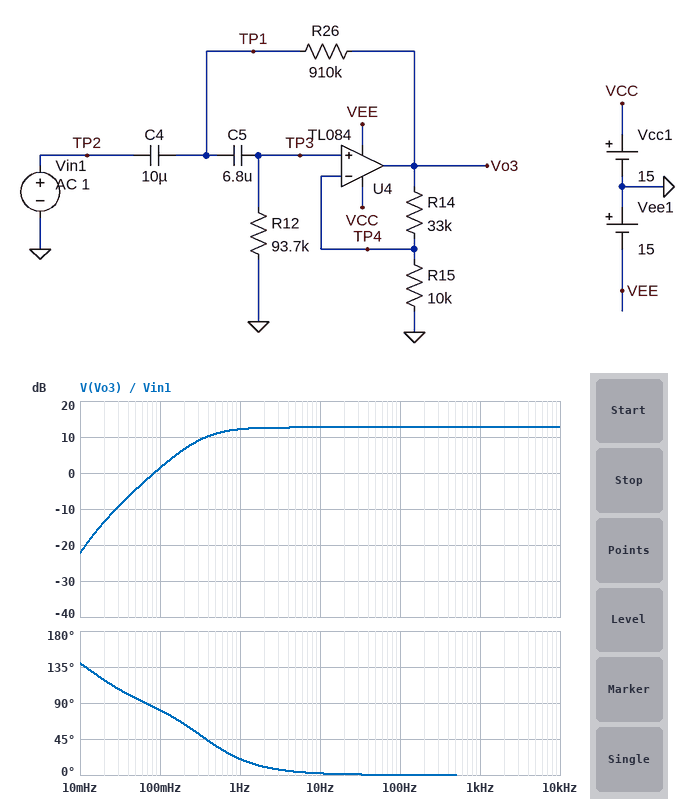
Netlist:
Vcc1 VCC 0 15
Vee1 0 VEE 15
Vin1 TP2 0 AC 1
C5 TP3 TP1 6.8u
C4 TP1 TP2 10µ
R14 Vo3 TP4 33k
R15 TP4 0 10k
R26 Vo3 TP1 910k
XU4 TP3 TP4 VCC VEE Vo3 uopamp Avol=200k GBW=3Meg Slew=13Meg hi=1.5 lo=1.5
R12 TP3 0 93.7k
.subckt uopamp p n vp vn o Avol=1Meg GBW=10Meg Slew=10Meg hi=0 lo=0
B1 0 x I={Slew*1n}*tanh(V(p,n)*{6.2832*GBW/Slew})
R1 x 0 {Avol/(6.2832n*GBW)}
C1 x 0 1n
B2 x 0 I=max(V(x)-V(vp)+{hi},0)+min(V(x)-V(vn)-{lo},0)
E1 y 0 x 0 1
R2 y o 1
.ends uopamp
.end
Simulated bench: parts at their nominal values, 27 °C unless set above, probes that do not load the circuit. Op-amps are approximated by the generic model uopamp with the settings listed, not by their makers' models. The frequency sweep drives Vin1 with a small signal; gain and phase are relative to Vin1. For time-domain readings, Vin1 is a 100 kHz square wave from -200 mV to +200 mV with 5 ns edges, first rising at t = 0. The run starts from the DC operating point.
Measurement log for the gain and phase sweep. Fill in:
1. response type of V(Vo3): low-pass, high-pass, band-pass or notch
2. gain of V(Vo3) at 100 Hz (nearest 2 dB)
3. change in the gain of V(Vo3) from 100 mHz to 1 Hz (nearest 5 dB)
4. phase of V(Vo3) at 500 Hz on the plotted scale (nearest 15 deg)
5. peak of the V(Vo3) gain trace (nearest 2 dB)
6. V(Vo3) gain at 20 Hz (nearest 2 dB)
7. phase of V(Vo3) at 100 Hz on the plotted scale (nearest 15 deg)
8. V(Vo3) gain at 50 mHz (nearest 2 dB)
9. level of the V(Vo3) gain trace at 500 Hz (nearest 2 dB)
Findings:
high-pass
12 dB
10 dB
0 deg
12 dB
12 dB
0 deg
-4 dB
12 dB
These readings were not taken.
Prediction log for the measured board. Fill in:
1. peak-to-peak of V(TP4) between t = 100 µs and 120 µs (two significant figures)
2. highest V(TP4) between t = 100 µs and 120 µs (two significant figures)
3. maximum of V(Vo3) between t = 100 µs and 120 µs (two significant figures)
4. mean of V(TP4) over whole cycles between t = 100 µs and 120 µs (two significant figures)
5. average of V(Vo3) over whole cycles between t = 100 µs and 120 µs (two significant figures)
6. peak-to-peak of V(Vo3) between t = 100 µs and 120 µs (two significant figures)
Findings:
400 mV
400 mV
1.7 V
200 mV
860 mV
1.7 V
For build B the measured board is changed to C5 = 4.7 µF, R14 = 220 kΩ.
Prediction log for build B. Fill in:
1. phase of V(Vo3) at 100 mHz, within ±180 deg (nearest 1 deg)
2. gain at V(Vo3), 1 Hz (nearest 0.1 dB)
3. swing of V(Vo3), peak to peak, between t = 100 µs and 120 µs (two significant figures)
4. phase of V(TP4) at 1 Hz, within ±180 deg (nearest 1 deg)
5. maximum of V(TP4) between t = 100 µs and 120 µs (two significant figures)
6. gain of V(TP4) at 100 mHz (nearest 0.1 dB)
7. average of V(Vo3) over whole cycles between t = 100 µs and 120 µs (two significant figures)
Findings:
76 deg
27.2 dB
8.9 V
8 deg
390 mV
-3.6 dB
4.6 V
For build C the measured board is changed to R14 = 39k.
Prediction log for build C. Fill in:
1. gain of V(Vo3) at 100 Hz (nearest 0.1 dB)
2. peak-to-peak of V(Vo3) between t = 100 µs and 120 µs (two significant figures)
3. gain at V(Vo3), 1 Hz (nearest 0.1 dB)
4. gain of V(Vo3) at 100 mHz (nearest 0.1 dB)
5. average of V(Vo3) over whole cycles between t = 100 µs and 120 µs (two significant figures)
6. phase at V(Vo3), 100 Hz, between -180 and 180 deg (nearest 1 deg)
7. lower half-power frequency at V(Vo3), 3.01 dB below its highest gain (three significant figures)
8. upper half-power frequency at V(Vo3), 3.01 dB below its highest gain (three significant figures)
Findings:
13.8 dB
2.0 V
13.3 dB
2.8 dB
980 mV
0 deg
339 mHz
612 kHz
